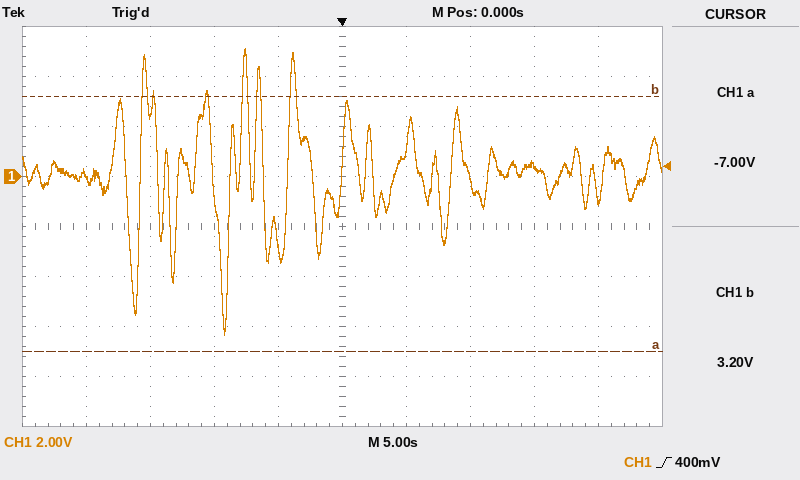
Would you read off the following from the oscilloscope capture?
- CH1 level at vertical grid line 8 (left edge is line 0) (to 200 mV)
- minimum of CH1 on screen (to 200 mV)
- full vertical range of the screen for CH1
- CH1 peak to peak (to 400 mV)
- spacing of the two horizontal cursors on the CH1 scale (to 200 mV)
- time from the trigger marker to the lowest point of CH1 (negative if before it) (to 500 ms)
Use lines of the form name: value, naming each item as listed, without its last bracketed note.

CH1 level at vertical grid line 8 (left edge is line 0): 400 mV
minimum of CH1 on screen: -6.4 V
full vertical range of the screen for CH1: 16 V
CH1 peak to peak: 11.6 V
spacing of the two horizontal cursors on the CH1 scale: 10.2 V
time from the trigger marker to the lowest point of CH1 (negative if before it): -9.0 s
